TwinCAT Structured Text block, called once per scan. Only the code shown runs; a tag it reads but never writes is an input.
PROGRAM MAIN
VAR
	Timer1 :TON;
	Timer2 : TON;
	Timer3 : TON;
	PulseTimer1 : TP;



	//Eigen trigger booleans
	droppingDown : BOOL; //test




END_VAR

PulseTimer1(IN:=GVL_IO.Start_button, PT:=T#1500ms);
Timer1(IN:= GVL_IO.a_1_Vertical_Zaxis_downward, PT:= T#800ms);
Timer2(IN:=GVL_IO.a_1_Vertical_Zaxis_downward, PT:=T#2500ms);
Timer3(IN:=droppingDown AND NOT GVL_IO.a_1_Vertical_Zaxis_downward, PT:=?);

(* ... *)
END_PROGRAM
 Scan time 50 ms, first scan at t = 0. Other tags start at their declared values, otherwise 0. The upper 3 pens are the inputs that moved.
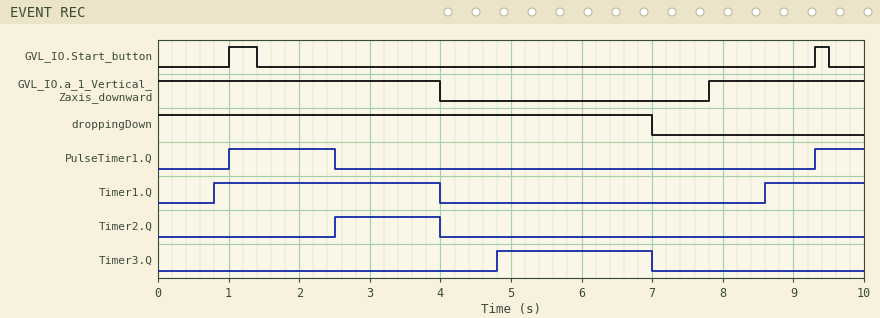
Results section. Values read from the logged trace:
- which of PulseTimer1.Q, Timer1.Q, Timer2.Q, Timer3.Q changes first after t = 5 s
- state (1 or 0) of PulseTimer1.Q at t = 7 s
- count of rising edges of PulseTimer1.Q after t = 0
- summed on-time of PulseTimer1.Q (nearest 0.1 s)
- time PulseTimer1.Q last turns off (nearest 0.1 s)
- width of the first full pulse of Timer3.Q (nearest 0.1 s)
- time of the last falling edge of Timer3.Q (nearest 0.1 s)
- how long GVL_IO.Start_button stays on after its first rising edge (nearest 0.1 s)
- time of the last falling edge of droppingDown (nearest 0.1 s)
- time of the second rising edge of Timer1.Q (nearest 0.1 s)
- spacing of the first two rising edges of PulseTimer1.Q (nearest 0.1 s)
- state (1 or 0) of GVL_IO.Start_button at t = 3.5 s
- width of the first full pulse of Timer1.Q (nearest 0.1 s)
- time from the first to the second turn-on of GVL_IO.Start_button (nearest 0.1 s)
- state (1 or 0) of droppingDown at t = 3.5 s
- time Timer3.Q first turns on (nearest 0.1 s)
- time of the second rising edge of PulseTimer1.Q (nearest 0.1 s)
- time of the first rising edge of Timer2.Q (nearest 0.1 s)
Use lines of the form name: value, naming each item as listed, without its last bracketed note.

which of PulseTimer1.Q, Timer1.Q, Timer2.Q, Timer3.Q changes first after t = 5 s: Timer3.Q
state (1 or 0) of PulseTimer1.Q at t = 7 s: 0
count of rising edges of PulseTimer1.Q after t = 0: 2
summed on-time of PulseTimer1.Q: 2.2 s
time PulseTimer1.Q last turns off: 2.5 s
width of the first full pulse of Timer3.Q: 2.2 s
time of the last falling edge of Timer3.Q: 7.0 s
how long GVL_IO.Start_button stays on after its first rising edge: 0.4 s
time of the last falling edge of droppingDown: 7.0 s
time of the second rising edge of Timer1.Q: 8.6 s
spacing of the first two rising edges of PulseTimer1.Q: 8.3 s
state (1 or 0) of GVL_IO.Start_button at t = 3.5 s: 0
width of the first full pulse of Timer1.Q: 3.2 s
time from the first to the second turn-on of GVL_IO.Start_button: 8.3 s
state (1 or 0) of droppingDown at t = 3.5 s: 1
time Timer3.Q first turns on: 4.8 s
time of the second rising edge of PulseTimer1.Q: 9.3 s
time of the first rising edge of Timer2.Q: 2.5 s
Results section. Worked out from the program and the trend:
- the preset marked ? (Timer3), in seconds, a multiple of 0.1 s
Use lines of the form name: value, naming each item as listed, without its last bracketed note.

the preset marked ? (Timer3), in seconds, a multiple of 0.1 s: 0.8 s
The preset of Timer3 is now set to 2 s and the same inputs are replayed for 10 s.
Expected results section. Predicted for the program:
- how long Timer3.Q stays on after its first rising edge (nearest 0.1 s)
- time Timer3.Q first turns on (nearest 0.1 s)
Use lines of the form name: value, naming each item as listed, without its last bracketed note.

how long Timer3.Q stays on after its first rising edge: 1.0 s
time Timer3.Q first turns on: 6.0 s
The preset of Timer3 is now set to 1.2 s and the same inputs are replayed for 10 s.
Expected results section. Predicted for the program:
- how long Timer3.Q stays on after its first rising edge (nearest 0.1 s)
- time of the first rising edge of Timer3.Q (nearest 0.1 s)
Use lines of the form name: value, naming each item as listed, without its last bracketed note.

how long Timer3.Q stays on after its first rising edge: 1.8 s
time of the first rising edge of Timer3.Q: 5.2 s
